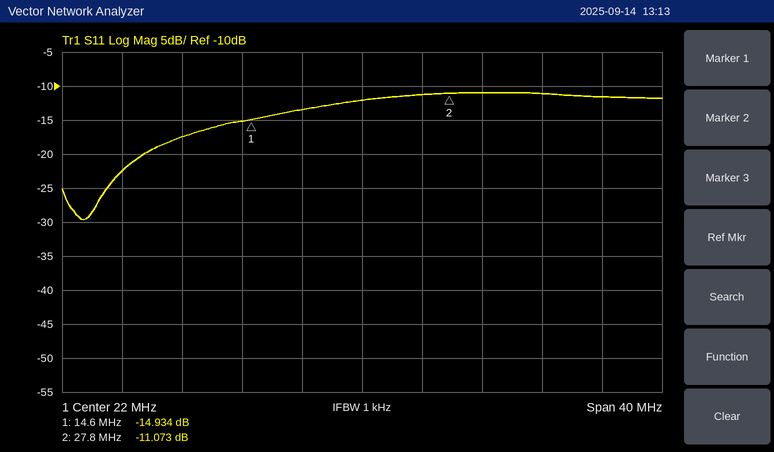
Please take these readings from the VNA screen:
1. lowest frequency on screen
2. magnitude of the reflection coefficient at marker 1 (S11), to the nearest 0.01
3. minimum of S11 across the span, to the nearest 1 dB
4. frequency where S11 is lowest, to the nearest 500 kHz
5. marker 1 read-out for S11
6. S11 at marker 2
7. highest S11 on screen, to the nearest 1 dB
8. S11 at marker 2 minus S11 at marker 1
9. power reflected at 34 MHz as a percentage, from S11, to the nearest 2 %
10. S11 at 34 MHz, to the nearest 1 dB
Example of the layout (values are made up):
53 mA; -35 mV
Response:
2 MHz; 0.18; -30 dB; 3.5 MHz; -14.934 dB; -11.073 dB; -11 dB; 3.861 dB; 8 %; -11 dB
